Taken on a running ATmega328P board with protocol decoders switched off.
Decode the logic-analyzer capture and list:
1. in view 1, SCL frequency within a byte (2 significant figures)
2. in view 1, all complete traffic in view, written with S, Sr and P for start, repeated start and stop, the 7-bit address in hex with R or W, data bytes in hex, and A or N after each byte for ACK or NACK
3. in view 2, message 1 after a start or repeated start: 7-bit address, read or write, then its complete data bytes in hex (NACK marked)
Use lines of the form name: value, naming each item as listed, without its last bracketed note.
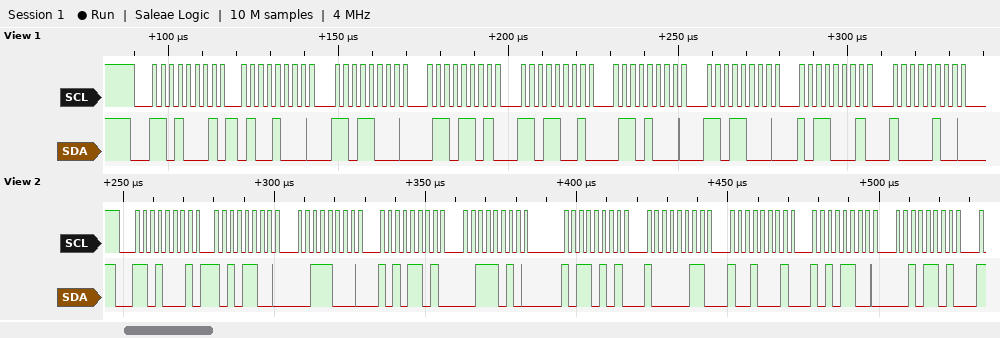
in view 1, SCL frequency within a byte: 400 kHz
in view 1, all complete traffic in view, written with S, Sr and P for start, repeated start and stop, the 7-bit address in hex with R or W, data bytes in hex, and A or N after each byte for ACK or NACK: S 68R A 48 A D8 A 6D A D9 A 68 A D8 A B1 A 84 A
in view 2, message 1 after a start or repeated start: 7-bit address, read or write, then its complete data bytes in hex: 0x68 read: AC 38 AD 3A B5 83 91 AC 2D
